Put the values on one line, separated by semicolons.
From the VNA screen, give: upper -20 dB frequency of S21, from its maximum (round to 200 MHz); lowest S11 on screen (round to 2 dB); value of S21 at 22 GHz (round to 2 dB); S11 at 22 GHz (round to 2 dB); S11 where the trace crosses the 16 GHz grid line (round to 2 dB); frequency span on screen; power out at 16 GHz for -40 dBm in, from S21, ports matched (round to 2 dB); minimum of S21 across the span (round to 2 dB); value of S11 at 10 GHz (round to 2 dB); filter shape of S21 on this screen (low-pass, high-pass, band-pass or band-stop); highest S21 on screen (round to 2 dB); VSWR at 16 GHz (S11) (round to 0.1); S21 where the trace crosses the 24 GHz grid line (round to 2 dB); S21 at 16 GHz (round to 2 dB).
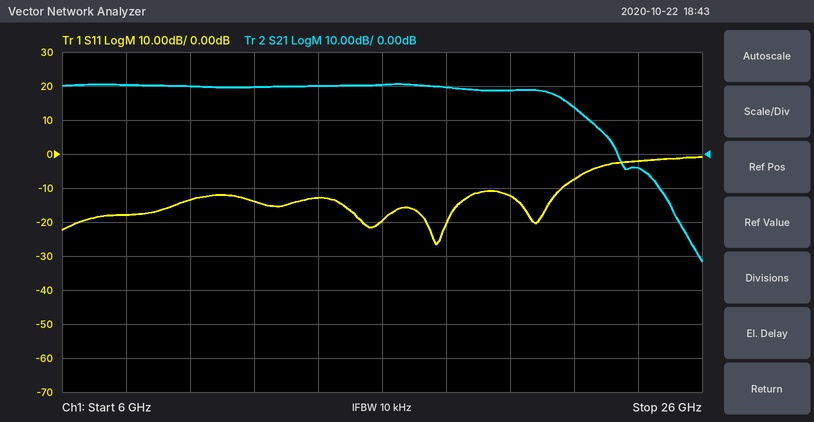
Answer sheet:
23.4 GHz; -26 dB; 14 dB; -8 dB; -20 dB; 20 GHz; -20 dBm; -32 dB; -14 dB; low-pass; 20 dB; 1.2; -4 dB; 20 dB
